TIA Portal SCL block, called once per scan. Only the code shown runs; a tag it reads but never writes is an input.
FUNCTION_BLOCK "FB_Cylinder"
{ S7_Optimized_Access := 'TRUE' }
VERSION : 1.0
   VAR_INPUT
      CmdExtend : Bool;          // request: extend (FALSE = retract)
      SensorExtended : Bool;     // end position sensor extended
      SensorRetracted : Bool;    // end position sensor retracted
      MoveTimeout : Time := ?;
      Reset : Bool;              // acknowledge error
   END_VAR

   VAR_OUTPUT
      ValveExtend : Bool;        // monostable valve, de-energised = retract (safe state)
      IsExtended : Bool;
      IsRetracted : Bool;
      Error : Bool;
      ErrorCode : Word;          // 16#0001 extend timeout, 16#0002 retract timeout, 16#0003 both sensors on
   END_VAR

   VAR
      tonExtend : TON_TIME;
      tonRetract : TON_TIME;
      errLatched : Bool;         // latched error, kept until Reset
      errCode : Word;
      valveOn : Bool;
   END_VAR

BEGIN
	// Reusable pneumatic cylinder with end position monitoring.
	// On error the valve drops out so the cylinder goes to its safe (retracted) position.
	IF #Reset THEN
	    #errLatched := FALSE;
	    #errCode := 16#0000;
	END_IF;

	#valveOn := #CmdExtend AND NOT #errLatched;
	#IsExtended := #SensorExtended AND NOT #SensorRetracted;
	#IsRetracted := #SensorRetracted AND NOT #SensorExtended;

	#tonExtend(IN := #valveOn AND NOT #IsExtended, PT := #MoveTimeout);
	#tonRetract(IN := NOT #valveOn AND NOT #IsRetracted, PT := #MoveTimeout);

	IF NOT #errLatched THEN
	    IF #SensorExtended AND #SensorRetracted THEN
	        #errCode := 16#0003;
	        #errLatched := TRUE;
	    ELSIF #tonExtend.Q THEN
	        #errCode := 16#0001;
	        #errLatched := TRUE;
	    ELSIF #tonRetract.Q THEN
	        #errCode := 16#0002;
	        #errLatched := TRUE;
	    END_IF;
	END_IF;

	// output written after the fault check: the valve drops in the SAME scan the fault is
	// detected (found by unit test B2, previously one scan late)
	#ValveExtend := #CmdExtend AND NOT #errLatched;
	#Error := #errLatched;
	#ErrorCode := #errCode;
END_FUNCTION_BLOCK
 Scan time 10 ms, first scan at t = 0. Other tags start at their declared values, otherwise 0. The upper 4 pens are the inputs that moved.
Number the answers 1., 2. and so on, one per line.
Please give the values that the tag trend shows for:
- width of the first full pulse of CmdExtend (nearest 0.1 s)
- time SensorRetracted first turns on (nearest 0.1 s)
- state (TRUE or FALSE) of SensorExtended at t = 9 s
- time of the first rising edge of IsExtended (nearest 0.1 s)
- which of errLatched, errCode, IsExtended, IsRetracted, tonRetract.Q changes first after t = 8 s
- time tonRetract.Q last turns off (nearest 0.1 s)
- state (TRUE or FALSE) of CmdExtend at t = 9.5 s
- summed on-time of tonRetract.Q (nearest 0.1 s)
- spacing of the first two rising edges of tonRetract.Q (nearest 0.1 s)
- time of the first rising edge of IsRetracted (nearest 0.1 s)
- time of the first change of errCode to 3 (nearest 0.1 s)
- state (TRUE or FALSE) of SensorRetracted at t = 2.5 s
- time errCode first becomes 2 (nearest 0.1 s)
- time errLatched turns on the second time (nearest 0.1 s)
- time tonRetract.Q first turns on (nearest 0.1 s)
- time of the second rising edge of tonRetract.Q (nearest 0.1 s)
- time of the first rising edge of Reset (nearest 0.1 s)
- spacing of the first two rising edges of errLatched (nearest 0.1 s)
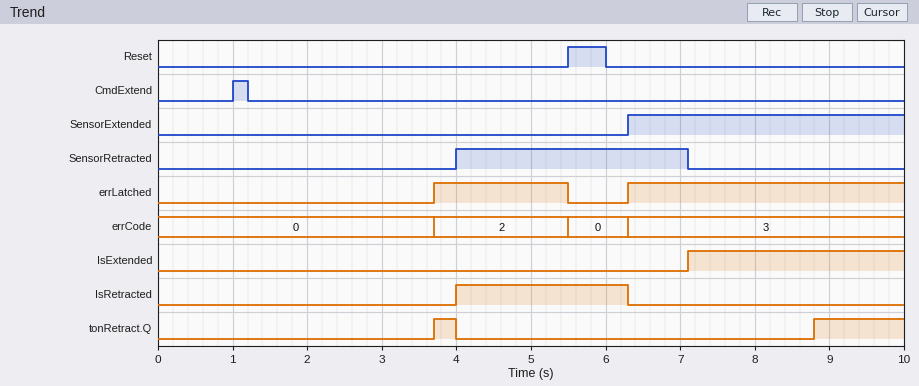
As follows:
1. 0.2 s
2. 4.0 s
3. TRUE
4. 7.1 s
5. tonRetract.Q
6. 4.0 s
7. FALSE
8. 1.5 s
9. 5.1 s
10. 4.0 s
11. 6.3 s
12. FALSE
13. 3.7 s
14. 6.3 s
15. 3.7 s
16. 8.8 s
17. 5.5 s
18. 2.6 s
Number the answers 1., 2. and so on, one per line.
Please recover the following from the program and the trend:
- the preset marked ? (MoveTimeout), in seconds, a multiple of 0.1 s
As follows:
1. 2.5 s
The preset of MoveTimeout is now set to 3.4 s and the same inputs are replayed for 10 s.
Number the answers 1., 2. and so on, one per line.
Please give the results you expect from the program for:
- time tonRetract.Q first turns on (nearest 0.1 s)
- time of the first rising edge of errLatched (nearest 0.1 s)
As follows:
1. 9.7 s
2. 6.3 s
